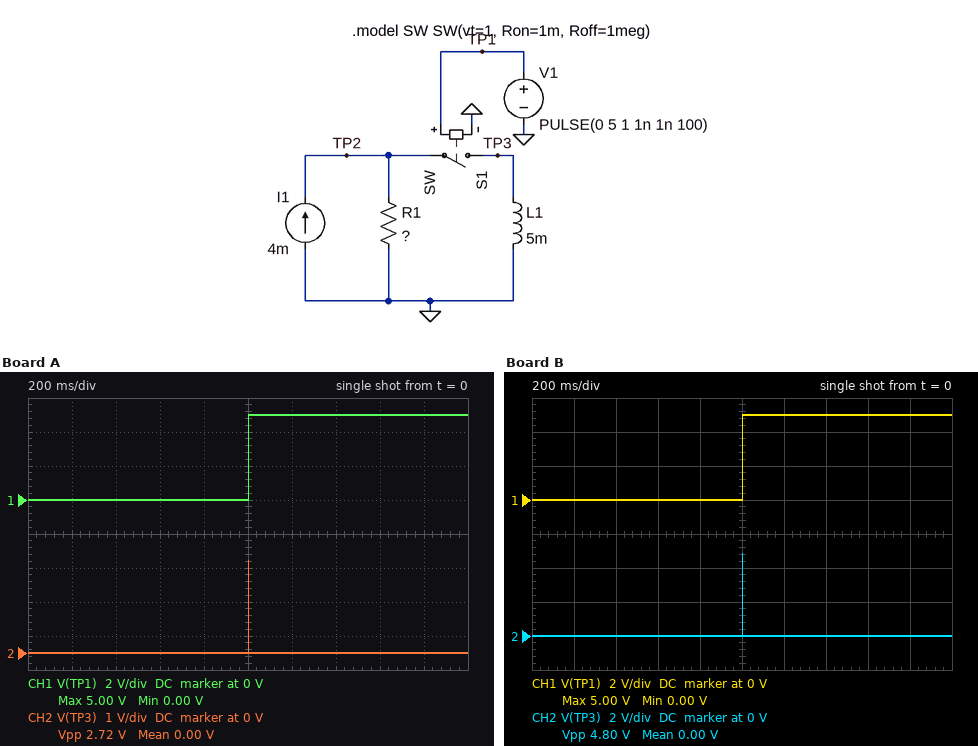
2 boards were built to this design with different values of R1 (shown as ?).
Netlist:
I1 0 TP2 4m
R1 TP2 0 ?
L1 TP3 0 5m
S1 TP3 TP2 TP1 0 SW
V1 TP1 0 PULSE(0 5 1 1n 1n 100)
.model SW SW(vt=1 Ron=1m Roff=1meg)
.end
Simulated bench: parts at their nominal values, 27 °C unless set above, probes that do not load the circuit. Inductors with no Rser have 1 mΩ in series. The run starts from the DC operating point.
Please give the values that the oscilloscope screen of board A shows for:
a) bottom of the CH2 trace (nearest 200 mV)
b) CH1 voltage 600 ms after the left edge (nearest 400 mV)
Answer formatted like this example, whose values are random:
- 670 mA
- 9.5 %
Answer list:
- 0 V
- 0 V
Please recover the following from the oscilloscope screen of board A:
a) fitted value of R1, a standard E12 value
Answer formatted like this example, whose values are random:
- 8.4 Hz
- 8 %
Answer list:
- 680 Ω
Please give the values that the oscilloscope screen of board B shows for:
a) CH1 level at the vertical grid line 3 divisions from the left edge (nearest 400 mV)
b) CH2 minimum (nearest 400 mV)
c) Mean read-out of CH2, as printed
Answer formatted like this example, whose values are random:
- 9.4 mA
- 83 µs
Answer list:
- 0 V
- 0 V
- 0.00 V
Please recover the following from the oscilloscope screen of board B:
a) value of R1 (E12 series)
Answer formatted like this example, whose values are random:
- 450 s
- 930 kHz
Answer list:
- 1.2 kΩ
